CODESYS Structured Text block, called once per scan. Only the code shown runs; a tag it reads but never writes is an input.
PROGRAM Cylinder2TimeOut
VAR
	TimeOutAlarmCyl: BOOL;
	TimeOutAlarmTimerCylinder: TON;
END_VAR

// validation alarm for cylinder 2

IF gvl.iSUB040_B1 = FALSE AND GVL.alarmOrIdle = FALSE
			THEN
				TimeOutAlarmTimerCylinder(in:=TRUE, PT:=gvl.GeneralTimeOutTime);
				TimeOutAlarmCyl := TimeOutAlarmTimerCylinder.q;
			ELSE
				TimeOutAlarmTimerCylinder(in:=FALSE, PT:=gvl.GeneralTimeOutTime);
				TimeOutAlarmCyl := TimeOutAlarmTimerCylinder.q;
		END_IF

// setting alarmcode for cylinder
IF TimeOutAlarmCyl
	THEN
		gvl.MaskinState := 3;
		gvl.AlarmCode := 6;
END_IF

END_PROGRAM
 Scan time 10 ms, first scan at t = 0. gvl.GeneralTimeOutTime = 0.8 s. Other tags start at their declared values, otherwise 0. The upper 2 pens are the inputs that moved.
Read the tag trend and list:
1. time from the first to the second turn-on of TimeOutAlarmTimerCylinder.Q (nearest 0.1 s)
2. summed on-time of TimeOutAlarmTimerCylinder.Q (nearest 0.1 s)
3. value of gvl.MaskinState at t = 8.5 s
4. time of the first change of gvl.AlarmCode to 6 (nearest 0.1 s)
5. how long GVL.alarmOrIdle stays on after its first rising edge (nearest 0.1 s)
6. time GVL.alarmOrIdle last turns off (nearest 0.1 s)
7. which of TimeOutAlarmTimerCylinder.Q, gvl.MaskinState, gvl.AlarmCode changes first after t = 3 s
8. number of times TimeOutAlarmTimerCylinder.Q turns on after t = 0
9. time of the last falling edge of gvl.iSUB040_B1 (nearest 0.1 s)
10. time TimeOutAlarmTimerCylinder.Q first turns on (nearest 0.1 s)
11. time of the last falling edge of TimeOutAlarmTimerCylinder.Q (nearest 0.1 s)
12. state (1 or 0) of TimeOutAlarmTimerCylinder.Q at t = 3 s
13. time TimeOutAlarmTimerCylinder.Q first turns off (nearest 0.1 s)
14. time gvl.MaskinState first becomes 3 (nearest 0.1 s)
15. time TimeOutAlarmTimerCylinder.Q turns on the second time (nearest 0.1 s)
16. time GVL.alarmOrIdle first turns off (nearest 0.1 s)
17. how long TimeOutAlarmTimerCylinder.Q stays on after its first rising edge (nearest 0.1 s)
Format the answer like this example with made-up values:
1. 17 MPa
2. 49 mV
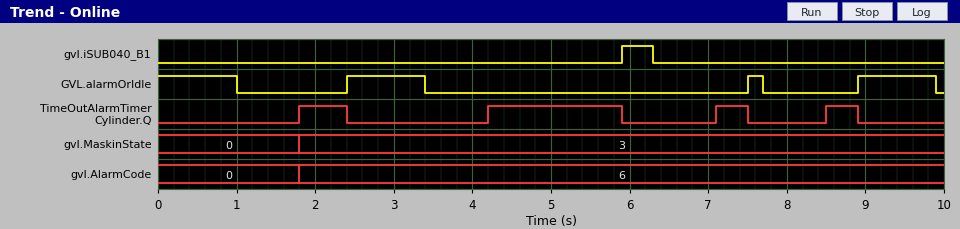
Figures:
1. 2.4 s
2. 3.1 s
3. 3
4. 1.8 s
5. 1.0 s
6. 9.9 s
7. TimeOutAlarmTimerCylinder.Q
8. 4
9. 6.3 s
10. 1.8 s
11. 8.9 s
12. 0
13. 2.4 s
14. 1.8 s
15. 4.2 s
16. 1.0 s
17. 0.6 s
